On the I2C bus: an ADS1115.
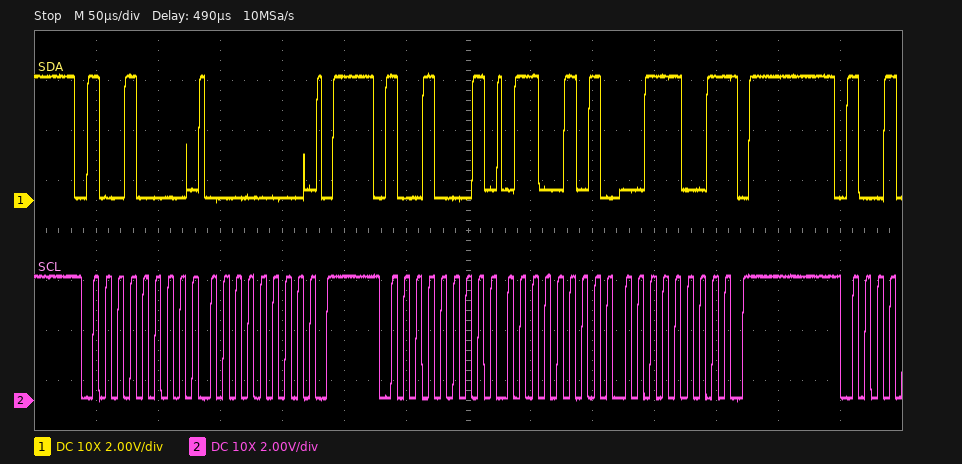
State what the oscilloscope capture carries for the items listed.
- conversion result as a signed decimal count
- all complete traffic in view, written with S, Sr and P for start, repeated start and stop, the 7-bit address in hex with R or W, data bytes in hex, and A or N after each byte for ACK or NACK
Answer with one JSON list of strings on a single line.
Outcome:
["25913", "S 48W A 00 A P S 48R A 65 A 39 N P"]
